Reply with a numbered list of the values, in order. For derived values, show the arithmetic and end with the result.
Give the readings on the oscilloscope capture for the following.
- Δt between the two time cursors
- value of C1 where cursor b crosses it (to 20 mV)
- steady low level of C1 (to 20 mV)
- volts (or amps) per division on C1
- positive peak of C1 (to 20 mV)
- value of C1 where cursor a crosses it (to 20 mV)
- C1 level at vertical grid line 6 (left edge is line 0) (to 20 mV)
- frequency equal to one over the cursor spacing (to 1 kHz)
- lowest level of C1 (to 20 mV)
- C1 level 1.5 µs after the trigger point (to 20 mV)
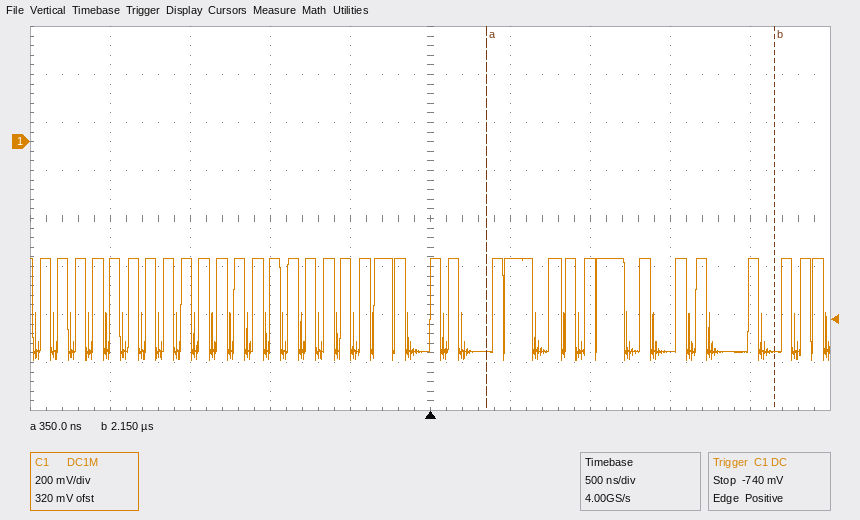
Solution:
1. 2.15 µs − (350 ns) = 1.80 µs
2. -880 mV
3. -880 mV
4. 200 mV
5. -480 mV
6. -880 mV
7. -480 mV
8. 1 / 1.80 µs ≈ 556 kHz
9. -920 mV
10. -880 mV
